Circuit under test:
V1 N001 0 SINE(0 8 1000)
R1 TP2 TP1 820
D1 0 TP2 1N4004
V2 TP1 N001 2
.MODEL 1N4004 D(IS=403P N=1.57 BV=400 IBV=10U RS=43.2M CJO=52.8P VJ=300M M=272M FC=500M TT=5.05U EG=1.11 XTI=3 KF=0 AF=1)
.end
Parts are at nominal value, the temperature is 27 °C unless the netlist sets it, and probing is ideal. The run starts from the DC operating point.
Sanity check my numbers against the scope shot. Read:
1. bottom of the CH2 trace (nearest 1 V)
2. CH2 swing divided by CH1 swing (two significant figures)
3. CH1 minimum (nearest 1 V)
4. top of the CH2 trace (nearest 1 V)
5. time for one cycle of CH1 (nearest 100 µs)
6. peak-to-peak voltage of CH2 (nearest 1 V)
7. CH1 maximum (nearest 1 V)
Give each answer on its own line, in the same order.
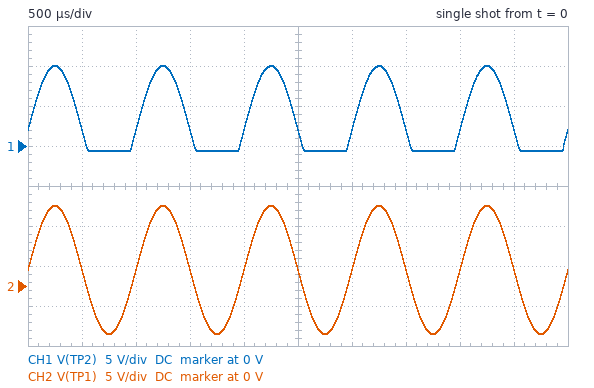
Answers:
-6 V
1.5
-1 V
10 V
1.0 ms
16 V
10 V
